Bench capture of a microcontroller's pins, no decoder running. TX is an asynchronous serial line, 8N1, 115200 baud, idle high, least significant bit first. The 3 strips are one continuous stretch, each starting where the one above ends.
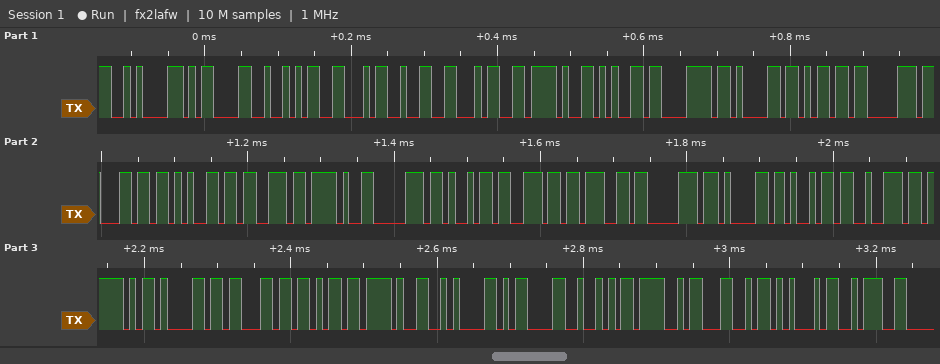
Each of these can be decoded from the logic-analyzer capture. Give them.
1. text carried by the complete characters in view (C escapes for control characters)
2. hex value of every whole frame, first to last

"\n\rRF24/examples/pingpair_ack/\n\rROLE:"
0A 0D 52 46 32 34 2F 65 78 61 6D 70 6C 65 73 2F 70 69 6E 67 70 61 69 72 5F 61 63 6B 2F 0A 0D 52 4F 4C 45 3A
